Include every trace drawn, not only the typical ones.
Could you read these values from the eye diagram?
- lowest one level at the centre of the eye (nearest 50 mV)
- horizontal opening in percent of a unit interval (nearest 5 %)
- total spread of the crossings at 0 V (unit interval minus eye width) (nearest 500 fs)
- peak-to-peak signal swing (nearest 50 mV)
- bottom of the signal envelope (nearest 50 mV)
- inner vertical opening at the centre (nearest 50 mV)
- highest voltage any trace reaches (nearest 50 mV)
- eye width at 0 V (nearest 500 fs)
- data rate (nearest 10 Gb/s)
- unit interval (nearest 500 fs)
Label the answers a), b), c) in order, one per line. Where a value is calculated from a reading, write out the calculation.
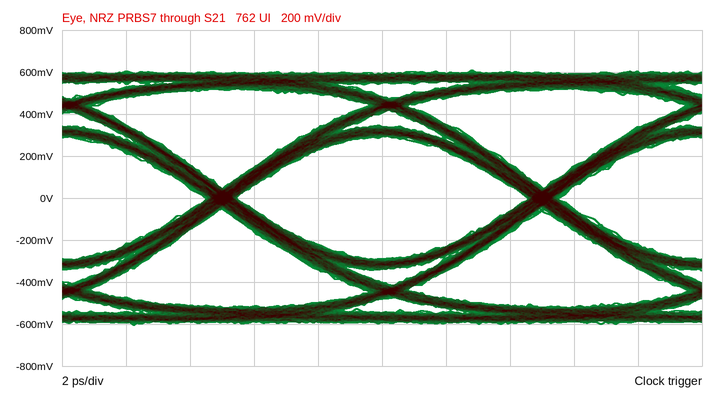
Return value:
a) 300 mV
b) 9.0 ps / 10.0 ps ≈ 90 %
c) 1.0 ps
d) 1.20 V
e) -600 mV
f) 600 mV
g) 600 mV
h) 9.0 ps
i) 100 Gb/s
j) 10.0 ps
